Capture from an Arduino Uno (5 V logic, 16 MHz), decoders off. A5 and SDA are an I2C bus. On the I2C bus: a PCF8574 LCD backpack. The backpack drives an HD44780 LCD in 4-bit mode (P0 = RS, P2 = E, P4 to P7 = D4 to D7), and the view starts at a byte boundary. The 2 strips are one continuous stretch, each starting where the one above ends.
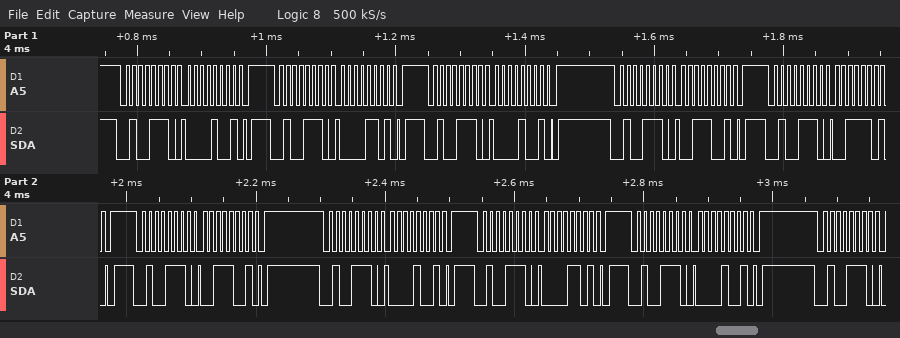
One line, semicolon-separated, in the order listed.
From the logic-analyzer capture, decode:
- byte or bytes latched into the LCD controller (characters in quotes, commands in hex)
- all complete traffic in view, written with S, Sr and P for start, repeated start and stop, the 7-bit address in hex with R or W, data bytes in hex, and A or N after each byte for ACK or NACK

data 0x03; S 27W A 09 A P S 27W A 0D A P S 27W A 09 A P S 27W A 39 A P S 27W A 3D A P S 27W A 39 A P S 27W A 09 A P S 27W A 0D A P S 27W A 09 A P S 27W A
